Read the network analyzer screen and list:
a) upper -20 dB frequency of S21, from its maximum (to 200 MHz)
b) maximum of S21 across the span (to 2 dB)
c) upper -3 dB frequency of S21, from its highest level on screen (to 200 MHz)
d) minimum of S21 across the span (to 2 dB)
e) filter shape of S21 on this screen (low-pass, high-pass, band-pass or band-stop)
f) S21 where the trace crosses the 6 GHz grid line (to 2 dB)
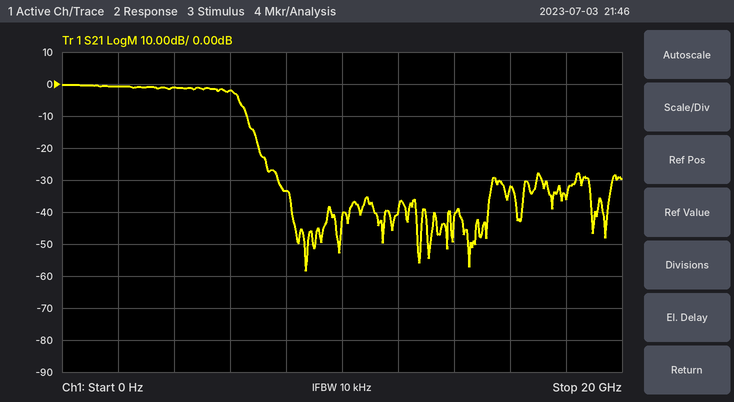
7.0 GHz
0 dB
6.2 GHz
-58 dB
low-pass
-2 dB
